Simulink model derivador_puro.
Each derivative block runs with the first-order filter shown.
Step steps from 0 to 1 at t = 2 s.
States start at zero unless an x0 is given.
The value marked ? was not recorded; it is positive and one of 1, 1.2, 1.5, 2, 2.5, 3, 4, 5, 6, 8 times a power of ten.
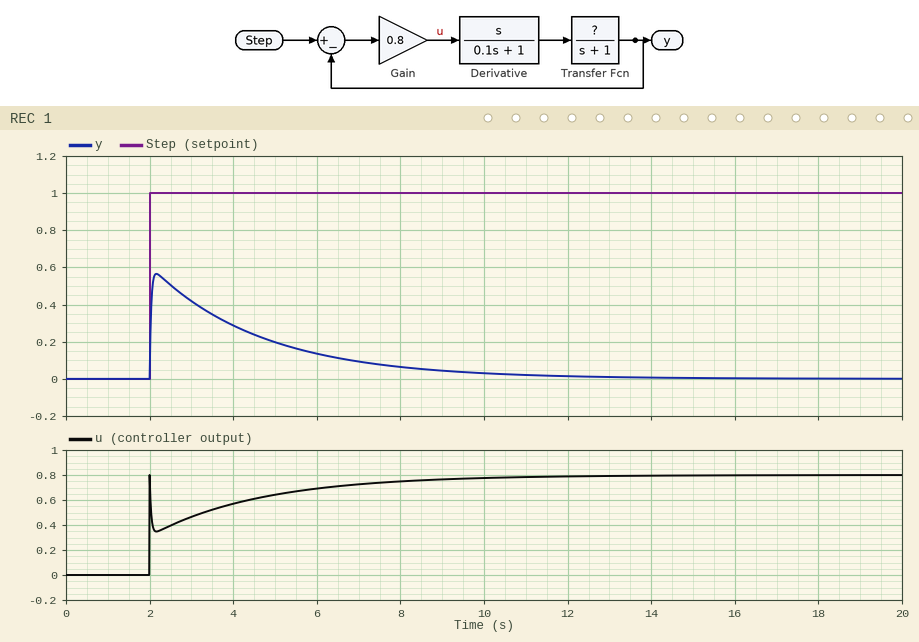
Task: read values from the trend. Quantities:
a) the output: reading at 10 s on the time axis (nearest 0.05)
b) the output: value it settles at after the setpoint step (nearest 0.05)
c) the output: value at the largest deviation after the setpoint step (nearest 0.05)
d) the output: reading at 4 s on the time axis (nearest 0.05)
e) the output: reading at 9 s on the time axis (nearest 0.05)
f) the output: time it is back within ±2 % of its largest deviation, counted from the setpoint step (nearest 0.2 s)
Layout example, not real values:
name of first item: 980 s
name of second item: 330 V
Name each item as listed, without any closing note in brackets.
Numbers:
the output: reading at 10 s on the time axis: 0.05
the output: value it settles at after the setpoint step: 0.00
the output: value at the largest deviation after the setpoint step: 0.55
the output: reading at 4 s on the time axis: 0.30
the output: reading at 9 s on the time axis: 0.05
the output: time it is back within ±2 % of its largest deviation, counted from the setpoint step: 10.6 s
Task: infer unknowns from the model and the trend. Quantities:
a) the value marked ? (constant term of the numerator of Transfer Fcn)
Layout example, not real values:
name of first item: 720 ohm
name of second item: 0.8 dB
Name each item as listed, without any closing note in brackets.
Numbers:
the value marked ?: 2
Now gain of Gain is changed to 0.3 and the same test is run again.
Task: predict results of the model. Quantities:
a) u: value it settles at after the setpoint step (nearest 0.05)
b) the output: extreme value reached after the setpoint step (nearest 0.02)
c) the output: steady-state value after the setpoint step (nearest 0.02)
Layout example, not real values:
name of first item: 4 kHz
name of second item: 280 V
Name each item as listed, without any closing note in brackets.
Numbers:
u: value it settles at after the setpoint step: 0.30
the output: extreme value reached after the setpoint step: 0.32
the output: steady-state value after the setpoint step: 0.00
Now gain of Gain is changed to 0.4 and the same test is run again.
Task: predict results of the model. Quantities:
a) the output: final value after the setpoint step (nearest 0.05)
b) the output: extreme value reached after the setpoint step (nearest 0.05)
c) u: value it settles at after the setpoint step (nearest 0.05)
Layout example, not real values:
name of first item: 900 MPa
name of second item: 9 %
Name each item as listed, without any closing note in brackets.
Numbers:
the output: final value after the setpoint step: 0.00
the output: extreme value reached after the setpoint step: 0.40
u: value it settles at after the setpoint step: 0.40
